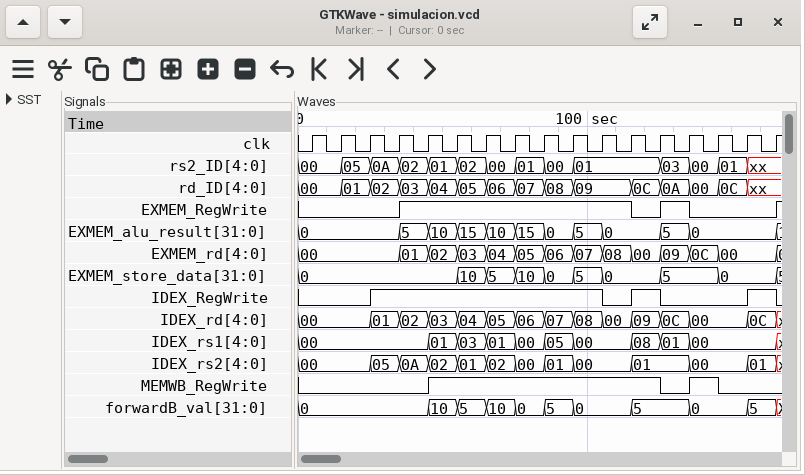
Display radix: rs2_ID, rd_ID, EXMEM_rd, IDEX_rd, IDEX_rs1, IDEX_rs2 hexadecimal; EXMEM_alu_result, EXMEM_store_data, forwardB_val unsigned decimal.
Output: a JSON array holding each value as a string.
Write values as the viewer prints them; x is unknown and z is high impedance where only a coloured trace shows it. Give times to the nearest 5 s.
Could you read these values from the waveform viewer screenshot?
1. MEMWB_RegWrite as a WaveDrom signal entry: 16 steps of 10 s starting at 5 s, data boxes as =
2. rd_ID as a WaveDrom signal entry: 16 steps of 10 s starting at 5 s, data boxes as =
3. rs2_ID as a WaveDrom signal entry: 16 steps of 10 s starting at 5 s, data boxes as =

["{name: 'MEMWB_RegWrite', wave: '0...1.......010.'}", "{name: 'rd_ID', wave: '==========.====x', data: '00 01 02 03 04 05 06 07 08 09 0C 0A 00 0C'}", "{name: 'rs2_ID', wave: '==========..===x', data: '00 05 0A 02 01 02 00 01 00 01 03 00 01'}"]
